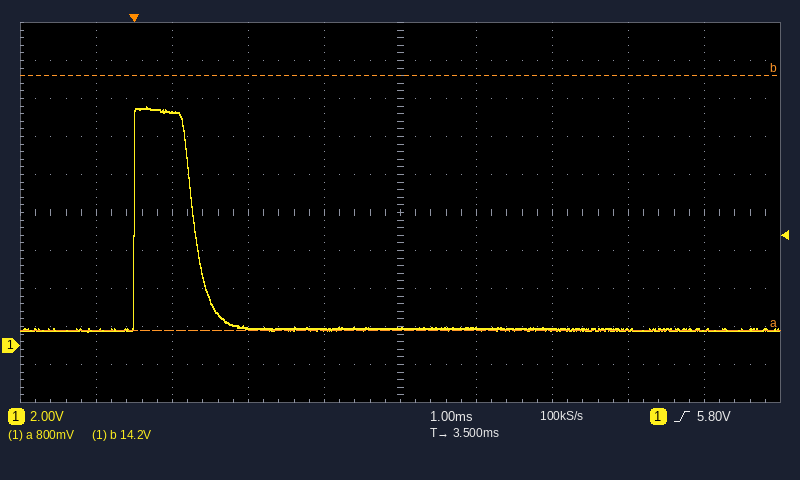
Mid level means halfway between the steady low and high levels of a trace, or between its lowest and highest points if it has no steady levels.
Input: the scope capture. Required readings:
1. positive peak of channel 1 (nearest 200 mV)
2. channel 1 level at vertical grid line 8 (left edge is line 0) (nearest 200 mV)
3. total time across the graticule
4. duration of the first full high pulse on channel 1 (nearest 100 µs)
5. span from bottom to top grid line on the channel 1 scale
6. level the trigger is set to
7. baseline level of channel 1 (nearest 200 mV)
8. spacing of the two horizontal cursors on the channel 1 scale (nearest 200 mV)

12.6 V
800 mV
10 ms
800 µs
20 V
5.80 V
800 mV
13.4 V
